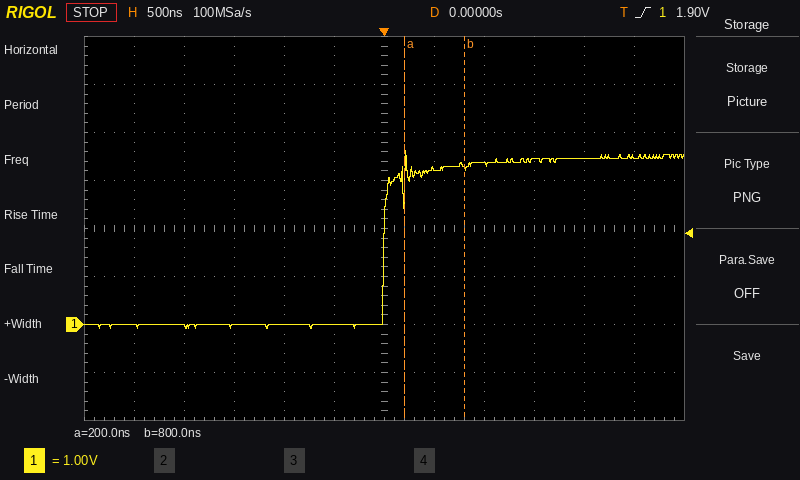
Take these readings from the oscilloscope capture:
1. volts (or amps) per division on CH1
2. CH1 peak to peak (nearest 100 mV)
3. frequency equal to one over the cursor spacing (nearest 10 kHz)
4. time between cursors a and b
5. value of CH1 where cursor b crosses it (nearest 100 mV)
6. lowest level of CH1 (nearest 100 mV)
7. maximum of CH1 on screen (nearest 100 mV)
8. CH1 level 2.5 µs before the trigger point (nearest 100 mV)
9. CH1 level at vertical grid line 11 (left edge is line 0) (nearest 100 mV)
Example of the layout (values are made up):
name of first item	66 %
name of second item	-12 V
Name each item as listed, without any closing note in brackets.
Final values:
volts (or amps) per division on CH1	1 V
CH1 peak to peak	3.7 V
frequency equal to one over the cursor spacing	1.67 MHz
time between cursors a and b	600 ns
value of CH1 where cursor b crosses it	3.3 V
lowest level of CH1	-100 mV
maximum of CH1 on screen	3.6 V
CH1 level 2.5 µs before the trigger point	0.0 V
CH1 level at vertical grid line 11 (left edge is line 0)	3.5 V
